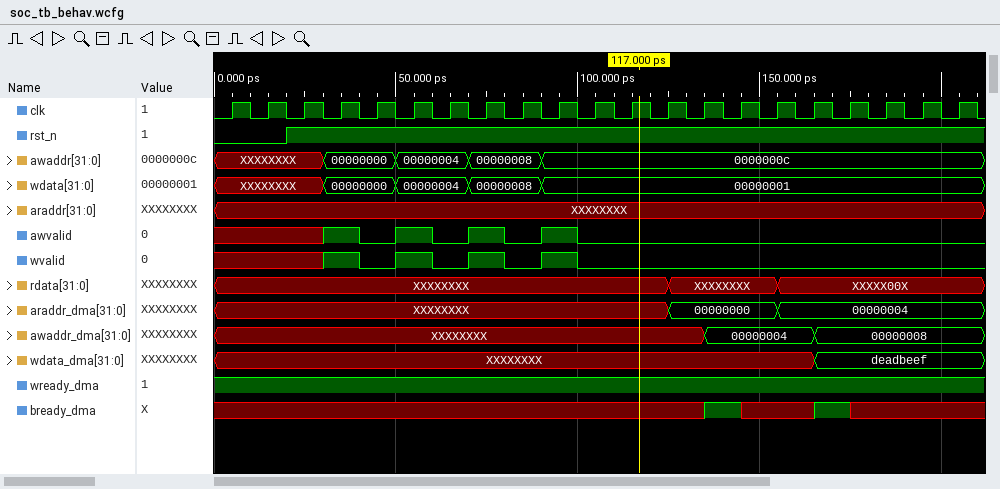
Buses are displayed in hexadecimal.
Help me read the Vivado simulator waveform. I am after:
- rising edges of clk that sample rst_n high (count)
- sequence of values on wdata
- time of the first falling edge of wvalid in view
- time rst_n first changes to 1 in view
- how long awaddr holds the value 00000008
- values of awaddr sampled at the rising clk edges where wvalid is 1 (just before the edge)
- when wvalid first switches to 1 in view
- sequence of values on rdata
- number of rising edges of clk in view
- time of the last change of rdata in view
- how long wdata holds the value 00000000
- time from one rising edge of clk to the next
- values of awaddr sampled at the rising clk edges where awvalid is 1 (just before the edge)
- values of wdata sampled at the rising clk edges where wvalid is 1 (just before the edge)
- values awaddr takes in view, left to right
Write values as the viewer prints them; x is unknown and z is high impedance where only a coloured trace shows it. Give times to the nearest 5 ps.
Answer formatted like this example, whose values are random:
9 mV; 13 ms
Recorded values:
19; XXXXXXXX, 00000000, 00000004, 00000008, 00000001; 40 ps; 20 ps; 20 ps; 00000000, 00000004, 00000008, 0000000c; 30 ps; XXXXXXXX, XXXXXXXX, XXXXX00X; 21; 155 ps; 20 ps; 10 ps; 00000000, 00000004, 00000008, 0000000c; 00000000, 00000004, 00000008, 00000001; XXXXXXXX, 00000000, 00000004, 00000008, 0000000c
